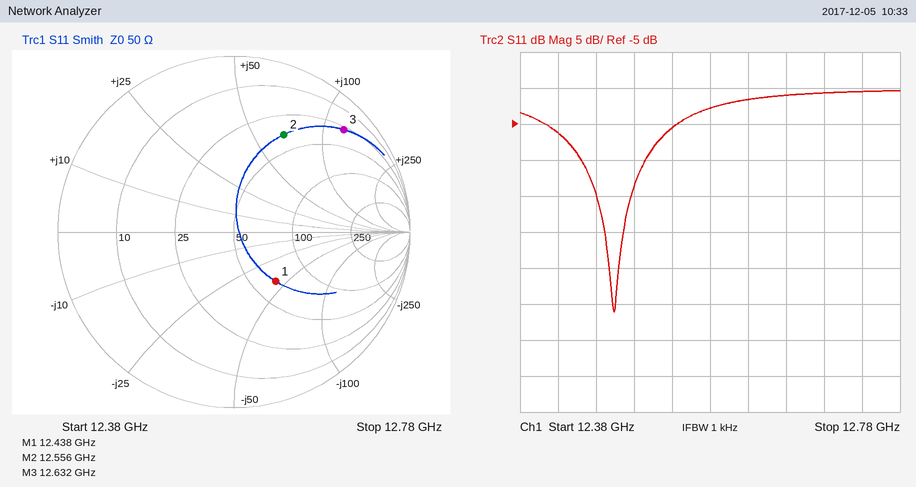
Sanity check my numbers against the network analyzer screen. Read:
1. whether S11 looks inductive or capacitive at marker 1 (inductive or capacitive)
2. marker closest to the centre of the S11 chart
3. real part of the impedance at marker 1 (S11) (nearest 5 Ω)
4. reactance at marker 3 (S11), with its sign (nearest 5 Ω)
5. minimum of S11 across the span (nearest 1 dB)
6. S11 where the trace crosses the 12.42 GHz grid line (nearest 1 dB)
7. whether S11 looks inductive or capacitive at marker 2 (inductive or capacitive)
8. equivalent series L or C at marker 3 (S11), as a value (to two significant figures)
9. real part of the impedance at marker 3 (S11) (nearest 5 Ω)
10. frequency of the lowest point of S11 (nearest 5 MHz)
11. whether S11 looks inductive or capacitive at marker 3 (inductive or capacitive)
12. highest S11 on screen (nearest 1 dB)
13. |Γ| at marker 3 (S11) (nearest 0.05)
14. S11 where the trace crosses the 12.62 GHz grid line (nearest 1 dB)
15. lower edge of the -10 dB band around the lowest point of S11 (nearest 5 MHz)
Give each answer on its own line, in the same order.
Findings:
capacitive
marker 1
65 Ω
+120 Ω
-31 dB
-6 dB
inductive
1.5 nH
30 Ω
12.480 GHz
inductive
0 dB
0.85
-2 dB
12.445 GHz
